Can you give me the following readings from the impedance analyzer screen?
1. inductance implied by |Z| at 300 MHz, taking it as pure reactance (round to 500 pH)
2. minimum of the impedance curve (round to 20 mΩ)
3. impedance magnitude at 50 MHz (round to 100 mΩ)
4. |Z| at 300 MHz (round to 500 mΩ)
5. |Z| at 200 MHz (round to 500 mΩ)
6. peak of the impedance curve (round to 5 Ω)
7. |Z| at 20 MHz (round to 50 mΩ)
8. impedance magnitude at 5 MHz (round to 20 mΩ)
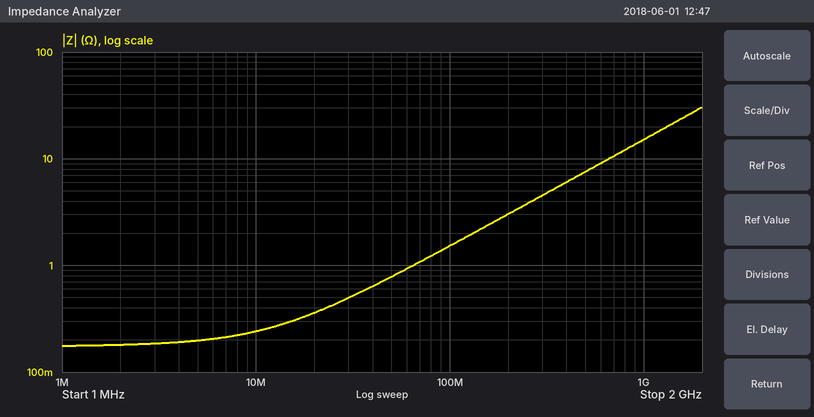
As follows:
2.5 nH
180 mΩ
800 mΩ
4.5 Ω
3.0 Ω
30 Ω
350 mΩ
200 mΩ
